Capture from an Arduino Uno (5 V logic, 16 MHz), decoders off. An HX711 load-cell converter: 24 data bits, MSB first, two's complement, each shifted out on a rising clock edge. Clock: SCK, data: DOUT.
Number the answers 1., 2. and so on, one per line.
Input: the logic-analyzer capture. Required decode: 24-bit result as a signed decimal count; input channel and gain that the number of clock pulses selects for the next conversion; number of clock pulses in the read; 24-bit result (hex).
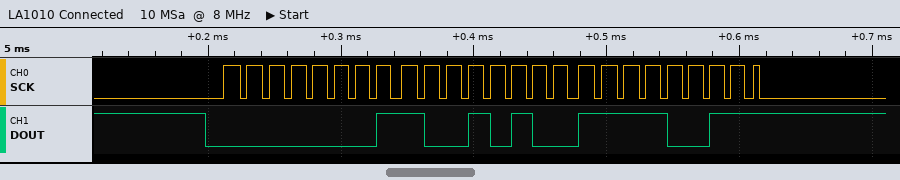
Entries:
1. 103667
2. channel A, gain 128
3. 25
4. 0x0194F3
